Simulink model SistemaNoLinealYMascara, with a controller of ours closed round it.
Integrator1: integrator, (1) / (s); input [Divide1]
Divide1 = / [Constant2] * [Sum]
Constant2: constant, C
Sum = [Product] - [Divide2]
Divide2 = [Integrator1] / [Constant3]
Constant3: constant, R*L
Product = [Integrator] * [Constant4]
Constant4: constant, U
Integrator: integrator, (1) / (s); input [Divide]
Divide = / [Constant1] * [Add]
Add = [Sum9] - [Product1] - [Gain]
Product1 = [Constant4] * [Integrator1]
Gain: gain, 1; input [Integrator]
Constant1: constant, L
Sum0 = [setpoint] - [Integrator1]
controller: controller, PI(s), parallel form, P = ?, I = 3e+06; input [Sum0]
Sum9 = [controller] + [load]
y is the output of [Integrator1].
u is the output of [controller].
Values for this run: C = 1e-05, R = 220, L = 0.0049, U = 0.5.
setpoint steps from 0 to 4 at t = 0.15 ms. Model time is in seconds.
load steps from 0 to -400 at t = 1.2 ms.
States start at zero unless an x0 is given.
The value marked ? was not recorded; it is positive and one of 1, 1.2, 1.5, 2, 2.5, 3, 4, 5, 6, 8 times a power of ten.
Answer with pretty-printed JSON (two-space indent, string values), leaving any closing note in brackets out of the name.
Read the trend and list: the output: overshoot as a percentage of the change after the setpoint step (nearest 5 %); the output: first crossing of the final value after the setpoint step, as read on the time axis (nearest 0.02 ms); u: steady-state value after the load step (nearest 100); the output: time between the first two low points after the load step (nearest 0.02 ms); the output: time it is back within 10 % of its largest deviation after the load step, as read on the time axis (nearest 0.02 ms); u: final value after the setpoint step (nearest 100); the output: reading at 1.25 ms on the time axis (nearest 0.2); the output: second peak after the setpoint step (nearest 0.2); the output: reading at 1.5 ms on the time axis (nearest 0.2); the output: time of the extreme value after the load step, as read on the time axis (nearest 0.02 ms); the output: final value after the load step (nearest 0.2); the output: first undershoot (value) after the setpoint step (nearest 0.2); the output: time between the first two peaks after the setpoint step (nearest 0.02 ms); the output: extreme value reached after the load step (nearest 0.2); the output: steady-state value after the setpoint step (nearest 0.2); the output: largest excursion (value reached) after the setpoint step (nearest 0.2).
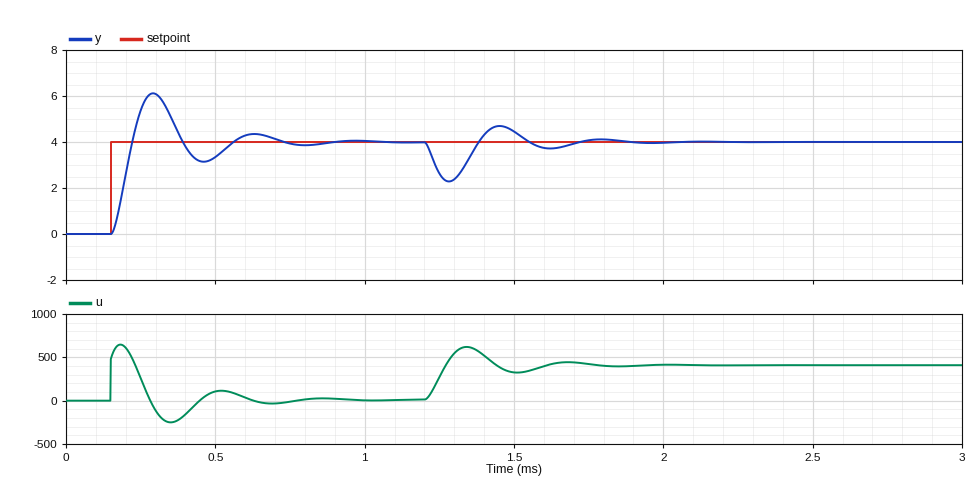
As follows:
{
  "the output: overshoot as a percentage of the change after the setpoint step": "55 %",
  "the output: first crossing of the final value after the setpoint step, as read on the time axis": "0.22 ms",
  "u: steady-state value after the load step": "400",
  "the output: time between the first two low points after the load step": "0.34 ms",
  "the output: time it is back within 10 % of its largest deviation after the load step, as read on the time axis": "1.68 ms",
  "u: final value after the setpoint step": "0",
  "the output: reading at 1.25 ms on the time axis": "2.6",
  "the output: second peak after the setpoint step": "4.4",
  "the output: reading at 1.5 ms on the time axis": "4.4",
  "the output: time of the extreme value after the load step, as read on the time axis": "1.28 ms",
  "the output: final value after the load step": "4.0",
  "the output: first undershoot (value) after the setpoint step": "3.2",
  "the output: time between the first two peaks after the setpoint step": "0.34 ms",
  "the output: extreme value reached after the load step": "2.2",
  "the output: steady-state value after the setpoint step": "4.0",
  "the output: largest excursion (value reached) after the setpoint step": "6.2"
}
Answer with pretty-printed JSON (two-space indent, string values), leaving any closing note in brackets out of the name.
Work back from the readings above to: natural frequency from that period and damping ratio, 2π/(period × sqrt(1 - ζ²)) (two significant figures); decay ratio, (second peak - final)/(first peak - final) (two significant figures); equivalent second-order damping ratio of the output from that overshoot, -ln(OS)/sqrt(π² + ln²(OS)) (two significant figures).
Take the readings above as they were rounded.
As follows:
{
  "natural frequency from that period and damping ratio, 2π/(period × sqrt(1 - ζ²))": "19 rad/ms",
  "decay ratio, (second peak - final)/(first peak - final)": "0.18",
  "equivalent second-order damping ratio of the output from that overshoot, -ln(OS)/sqrt(π² + ln²(OS))": "0.19"
}
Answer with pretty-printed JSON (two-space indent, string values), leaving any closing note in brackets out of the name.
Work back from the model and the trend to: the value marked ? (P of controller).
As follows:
{
  "the value marked ?": "120"
}
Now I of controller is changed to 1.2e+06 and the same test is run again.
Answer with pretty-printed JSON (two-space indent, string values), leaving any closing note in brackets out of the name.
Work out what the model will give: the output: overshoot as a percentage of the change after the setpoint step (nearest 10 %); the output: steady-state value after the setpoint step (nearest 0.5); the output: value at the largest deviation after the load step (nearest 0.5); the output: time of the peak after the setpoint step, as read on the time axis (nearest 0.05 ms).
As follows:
{
  "the output: overshoot as a percentage of the change after the setpoint step": "30 %",
  "the output: steady-state value after the setpoint step": "4.0",
  "the output: value at the largest deviation after the load step": "2.0",
  "the output: time of the peak after the setpoint step, as read on the time axis": "0.35 ms"
}
